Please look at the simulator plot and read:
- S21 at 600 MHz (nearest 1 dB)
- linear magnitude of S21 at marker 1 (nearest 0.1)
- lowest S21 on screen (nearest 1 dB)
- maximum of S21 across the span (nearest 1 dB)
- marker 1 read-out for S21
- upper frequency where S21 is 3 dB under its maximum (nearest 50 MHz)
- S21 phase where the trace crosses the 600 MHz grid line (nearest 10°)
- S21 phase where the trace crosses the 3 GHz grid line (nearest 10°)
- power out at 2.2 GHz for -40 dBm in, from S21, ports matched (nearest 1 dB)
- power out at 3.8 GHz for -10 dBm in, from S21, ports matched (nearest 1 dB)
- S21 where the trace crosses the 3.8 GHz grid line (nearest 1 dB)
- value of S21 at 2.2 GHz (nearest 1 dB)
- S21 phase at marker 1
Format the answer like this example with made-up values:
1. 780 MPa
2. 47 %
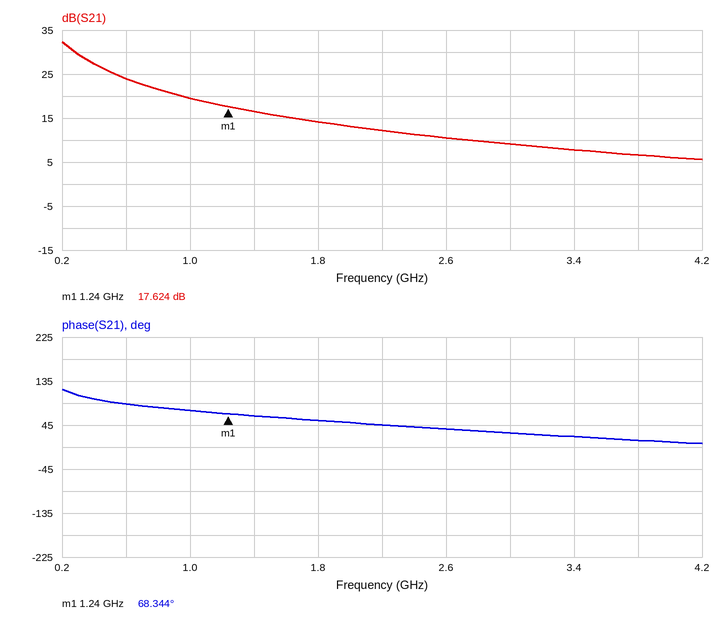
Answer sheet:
1. 24 dB
2. 7.6
3. 6 dB
4. 32 dB
5. 17.624 dB
6. 300 MHz
7. 90°
8. 30°
9. -28 dBm
10. -3 dBm
11. 7 dB
12. 12 dB
13. 68.344°
